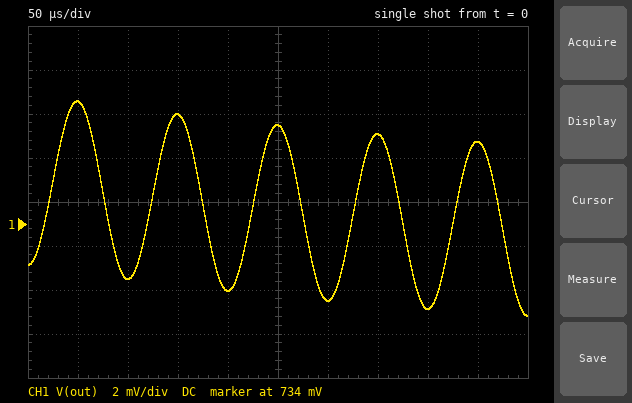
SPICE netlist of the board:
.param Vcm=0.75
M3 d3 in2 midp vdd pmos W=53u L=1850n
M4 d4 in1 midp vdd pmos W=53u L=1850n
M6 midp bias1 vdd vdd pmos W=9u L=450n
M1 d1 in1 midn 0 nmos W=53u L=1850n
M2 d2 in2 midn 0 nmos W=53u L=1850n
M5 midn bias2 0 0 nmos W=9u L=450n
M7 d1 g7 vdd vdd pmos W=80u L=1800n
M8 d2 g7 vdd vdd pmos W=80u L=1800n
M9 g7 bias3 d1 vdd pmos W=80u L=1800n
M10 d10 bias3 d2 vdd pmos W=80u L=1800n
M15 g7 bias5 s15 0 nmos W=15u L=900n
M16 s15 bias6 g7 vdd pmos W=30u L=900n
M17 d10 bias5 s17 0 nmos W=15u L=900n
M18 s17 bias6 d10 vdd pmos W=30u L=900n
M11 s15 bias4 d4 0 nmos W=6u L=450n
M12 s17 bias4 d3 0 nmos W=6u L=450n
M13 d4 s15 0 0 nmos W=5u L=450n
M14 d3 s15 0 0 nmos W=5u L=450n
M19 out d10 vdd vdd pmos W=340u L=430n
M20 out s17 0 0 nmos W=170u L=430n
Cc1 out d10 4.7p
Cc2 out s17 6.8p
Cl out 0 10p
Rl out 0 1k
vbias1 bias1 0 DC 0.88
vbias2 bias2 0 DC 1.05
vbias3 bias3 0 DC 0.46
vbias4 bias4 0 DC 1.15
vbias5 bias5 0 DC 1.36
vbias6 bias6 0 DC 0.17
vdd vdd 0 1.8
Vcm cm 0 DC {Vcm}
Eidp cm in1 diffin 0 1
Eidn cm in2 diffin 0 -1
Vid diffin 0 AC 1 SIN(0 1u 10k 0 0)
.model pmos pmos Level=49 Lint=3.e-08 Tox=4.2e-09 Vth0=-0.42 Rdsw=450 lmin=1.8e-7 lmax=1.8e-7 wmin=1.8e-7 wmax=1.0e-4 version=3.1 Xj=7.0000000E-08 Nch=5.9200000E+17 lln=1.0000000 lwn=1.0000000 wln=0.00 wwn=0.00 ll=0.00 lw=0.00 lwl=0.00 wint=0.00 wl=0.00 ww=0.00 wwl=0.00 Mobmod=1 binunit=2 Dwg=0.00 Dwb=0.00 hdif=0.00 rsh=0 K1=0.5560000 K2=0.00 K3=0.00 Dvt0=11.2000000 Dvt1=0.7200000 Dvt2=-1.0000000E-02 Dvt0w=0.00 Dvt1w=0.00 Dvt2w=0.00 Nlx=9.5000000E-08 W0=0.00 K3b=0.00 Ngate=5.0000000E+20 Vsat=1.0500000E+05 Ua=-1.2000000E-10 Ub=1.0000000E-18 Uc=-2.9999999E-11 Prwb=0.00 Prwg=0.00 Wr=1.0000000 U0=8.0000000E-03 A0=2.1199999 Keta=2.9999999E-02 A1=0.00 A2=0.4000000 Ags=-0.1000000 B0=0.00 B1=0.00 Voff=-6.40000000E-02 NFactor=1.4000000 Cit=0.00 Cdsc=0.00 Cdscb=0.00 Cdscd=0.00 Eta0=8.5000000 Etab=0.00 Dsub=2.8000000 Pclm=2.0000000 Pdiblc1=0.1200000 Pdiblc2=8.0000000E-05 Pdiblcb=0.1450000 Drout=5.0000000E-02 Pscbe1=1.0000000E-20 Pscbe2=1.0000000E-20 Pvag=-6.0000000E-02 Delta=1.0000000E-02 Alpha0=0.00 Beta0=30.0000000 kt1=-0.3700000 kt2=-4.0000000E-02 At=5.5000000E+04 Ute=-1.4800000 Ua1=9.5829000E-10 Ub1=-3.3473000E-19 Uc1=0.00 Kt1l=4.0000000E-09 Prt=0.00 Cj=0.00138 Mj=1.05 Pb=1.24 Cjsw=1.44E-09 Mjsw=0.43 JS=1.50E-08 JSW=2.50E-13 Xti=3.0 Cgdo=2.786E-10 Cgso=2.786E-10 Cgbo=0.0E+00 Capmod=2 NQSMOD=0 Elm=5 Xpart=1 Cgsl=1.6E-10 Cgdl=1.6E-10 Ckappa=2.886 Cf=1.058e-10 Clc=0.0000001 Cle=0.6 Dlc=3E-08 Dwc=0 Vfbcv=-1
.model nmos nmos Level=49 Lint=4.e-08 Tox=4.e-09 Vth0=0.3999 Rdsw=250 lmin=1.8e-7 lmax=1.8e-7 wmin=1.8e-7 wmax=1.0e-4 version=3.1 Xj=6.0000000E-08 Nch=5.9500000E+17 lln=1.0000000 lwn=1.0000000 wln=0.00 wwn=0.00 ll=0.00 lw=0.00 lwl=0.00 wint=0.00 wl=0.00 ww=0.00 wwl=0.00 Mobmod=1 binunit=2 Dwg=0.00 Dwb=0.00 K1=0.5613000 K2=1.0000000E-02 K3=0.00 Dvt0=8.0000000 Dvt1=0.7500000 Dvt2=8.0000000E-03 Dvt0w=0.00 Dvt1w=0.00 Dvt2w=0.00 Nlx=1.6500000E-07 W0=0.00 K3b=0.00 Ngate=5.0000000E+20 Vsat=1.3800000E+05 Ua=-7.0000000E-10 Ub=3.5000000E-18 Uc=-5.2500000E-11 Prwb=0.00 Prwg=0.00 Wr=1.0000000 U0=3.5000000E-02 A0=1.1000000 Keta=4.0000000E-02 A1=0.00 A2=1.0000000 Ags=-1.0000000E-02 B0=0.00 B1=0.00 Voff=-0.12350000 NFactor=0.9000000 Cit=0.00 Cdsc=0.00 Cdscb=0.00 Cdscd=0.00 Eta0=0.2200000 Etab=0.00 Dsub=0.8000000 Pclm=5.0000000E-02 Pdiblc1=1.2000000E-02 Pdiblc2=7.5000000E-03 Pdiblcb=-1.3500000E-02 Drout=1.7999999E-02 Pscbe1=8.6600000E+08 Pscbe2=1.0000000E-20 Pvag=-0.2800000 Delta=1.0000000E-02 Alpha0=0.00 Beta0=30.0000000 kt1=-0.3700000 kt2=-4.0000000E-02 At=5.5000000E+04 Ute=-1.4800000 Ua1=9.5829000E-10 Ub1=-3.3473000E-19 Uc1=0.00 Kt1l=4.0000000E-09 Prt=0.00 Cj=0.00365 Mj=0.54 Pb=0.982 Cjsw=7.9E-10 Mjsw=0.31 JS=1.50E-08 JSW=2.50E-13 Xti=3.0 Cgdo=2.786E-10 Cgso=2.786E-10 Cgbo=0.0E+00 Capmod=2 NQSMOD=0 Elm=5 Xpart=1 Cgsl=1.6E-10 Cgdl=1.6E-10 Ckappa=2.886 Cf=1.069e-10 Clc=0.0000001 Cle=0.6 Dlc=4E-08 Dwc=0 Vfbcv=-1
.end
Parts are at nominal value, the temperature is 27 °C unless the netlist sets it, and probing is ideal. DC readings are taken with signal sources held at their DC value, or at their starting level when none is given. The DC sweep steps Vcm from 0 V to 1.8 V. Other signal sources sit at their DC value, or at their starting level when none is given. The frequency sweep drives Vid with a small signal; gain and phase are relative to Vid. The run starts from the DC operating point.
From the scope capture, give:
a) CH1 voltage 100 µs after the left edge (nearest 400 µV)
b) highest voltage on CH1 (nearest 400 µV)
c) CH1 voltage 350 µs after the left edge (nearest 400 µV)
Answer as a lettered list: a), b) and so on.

a) 731.6 mV
b) 739.6 mV
c) 738.0 mV
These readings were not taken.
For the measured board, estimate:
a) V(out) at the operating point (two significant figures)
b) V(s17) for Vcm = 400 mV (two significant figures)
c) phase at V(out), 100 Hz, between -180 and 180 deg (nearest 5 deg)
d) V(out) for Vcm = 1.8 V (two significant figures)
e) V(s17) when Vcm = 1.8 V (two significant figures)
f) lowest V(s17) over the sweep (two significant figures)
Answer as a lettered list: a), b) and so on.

a) 730 mV
b) 790 mV
c) -20 deg
d) 1.7 V
e) 630 mV
f) 630 mV
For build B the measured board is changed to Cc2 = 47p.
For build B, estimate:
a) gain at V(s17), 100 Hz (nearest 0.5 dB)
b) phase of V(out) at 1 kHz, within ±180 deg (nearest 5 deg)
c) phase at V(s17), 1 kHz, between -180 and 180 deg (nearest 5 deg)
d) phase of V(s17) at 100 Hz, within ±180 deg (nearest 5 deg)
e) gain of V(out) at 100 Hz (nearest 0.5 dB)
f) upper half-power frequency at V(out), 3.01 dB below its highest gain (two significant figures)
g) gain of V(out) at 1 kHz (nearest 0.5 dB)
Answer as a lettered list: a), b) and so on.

a) 74.0 dB
b) -85 deg
c) 95 deg
d) 125 deg
e) 97.5 dB
f) 65 Hz
g) 79.0 dB
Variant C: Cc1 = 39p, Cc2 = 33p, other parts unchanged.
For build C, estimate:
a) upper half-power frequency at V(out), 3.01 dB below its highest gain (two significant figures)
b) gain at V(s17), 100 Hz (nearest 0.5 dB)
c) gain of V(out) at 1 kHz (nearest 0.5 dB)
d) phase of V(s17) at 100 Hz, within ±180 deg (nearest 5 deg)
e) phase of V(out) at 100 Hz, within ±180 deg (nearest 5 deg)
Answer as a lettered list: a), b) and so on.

a) 47 Hz
b) 72.0 dB
c) 76.0 dB
d) 115 deg
e) -65 deg
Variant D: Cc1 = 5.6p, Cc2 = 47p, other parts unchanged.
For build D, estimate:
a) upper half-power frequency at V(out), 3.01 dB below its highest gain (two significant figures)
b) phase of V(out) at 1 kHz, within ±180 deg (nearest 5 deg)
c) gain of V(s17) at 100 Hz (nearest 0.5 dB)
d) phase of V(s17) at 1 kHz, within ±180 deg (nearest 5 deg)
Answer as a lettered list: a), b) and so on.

a) 64 Hz
b) -85 deg
c) 74.0 dB
d) 95 deg
